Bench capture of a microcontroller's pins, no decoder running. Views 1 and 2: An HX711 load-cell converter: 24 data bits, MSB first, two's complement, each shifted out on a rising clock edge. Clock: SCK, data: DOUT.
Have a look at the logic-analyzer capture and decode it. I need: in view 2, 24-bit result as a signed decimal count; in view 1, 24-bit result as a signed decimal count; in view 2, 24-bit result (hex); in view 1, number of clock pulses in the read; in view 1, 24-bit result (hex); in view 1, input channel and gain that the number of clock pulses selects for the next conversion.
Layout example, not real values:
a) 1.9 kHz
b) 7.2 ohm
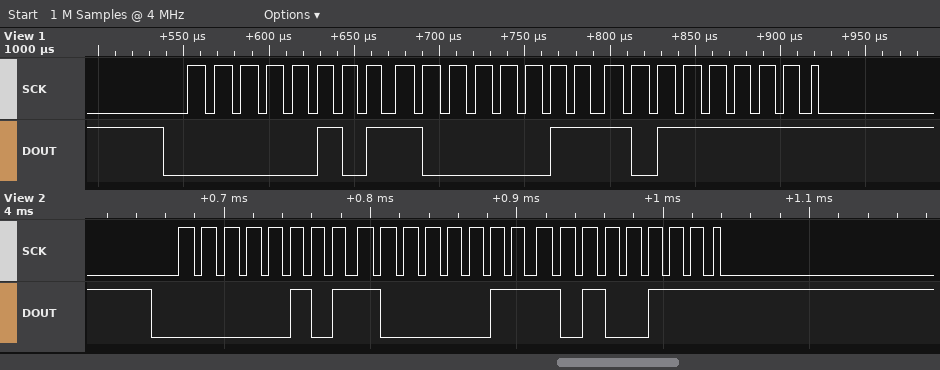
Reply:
a) 361383
b) 361407
c) 0x0583A7
d) 25
e) 0x0583BF
f) channel A, gain 128
